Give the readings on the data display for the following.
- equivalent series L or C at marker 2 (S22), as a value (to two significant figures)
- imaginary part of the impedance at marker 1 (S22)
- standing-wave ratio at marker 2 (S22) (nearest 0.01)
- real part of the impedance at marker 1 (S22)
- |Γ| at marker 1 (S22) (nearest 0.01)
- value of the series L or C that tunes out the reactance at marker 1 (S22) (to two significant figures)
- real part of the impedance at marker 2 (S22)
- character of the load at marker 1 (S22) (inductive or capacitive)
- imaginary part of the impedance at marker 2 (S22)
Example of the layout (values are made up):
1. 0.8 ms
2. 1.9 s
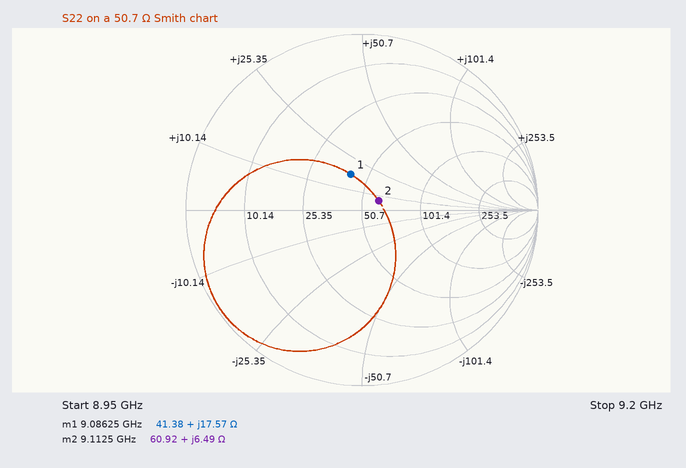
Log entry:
1. 110 pH
2. +17.57 Ω
3. 1.24
4. 41.38 Ω
5. 0.21
6. 1.00 pF
7. 60.92 Ω
8. inductive
9. +6.49 Ω
